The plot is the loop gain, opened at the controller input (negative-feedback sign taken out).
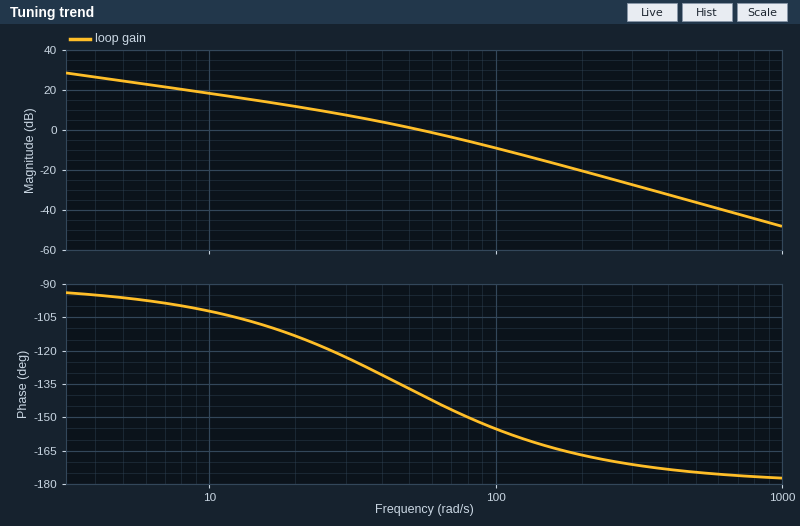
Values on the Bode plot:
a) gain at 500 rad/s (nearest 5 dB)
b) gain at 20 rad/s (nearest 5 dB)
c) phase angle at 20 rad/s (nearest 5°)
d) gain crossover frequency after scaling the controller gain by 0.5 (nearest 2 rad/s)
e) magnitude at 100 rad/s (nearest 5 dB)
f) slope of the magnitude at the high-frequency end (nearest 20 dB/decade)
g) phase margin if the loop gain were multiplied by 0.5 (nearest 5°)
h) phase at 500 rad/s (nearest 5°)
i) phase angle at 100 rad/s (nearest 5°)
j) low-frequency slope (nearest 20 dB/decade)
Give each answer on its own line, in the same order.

-35 dB
10 dB
-115°
34 rad/s
-10 dB
-40 dB/decade
55°
-175°
-155°
-20 dB/decade
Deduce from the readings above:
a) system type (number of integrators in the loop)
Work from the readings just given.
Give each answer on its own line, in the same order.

1
